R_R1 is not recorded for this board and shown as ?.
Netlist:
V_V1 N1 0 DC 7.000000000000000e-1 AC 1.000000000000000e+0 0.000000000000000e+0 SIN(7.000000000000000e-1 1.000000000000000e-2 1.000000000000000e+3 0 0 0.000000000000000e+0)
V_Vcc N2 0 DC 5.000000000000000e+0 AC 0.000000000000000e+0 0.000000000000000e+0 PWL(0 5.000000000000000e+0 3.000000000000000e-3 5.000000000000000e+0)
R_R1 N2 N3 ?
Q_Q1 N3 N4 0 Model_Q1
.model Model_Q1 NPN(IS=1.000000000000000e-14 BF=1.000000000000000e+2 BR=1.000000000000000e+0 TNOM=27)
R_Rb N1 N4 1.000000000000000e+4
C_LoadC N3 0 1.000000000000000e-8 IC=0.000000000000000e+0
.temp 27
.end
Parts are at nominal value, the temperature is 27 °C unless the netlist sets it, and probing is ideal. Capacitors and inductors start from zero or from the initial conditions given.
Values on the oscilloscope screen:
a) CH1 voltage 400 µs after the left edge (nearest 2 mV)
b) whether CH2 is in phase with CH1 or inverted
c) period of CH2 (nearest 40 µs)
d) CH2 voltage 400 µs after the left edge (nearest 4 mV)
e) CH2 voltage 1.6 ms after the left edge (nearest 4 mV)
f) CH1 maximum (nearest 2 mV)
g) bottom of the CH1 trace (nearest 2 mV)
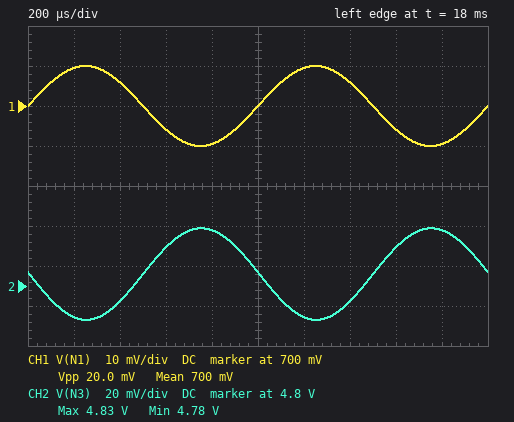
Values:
706 mV
inverted
1.00 ms
4.792 V
4.820 V
710 mV
690 mV
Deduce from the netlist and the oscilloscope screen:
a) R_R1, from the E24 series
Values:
330 Ω
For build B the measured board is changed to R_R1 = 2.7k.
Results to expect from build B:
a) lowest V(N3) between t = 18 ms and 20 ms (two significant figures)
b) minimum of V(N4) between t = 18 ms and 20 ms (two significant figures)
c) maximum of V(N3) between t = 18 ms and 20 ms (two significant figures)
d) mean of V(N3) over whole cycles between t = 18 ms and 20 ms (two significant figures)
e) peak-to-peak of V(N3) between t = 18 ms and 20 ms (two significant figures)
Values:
3.2 V
640 mV
3.6 V
3.4 V
370 mV
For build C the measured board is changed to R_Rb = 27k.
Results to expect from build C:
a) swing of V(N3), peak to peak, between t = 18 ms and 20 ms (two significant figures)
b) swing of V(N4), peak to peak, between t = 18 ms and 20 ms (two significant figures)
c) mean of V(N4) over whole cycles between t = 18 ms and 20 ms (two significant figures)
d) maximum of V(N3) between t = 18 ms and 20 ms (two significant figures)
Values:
18 mV
5.0 mV
620 mV
4.9 V
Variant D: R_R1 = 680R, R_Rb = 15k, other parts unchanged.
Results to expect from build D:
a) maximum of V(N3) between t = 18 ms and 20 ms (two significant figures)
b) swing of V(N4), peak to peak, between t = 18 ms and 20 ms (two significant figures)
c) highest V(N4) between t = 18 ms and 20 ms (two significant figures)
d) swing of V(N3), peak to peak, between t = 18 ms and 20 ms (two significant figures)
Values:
4.7 V
5.6 mV
640 mV
65 mV
